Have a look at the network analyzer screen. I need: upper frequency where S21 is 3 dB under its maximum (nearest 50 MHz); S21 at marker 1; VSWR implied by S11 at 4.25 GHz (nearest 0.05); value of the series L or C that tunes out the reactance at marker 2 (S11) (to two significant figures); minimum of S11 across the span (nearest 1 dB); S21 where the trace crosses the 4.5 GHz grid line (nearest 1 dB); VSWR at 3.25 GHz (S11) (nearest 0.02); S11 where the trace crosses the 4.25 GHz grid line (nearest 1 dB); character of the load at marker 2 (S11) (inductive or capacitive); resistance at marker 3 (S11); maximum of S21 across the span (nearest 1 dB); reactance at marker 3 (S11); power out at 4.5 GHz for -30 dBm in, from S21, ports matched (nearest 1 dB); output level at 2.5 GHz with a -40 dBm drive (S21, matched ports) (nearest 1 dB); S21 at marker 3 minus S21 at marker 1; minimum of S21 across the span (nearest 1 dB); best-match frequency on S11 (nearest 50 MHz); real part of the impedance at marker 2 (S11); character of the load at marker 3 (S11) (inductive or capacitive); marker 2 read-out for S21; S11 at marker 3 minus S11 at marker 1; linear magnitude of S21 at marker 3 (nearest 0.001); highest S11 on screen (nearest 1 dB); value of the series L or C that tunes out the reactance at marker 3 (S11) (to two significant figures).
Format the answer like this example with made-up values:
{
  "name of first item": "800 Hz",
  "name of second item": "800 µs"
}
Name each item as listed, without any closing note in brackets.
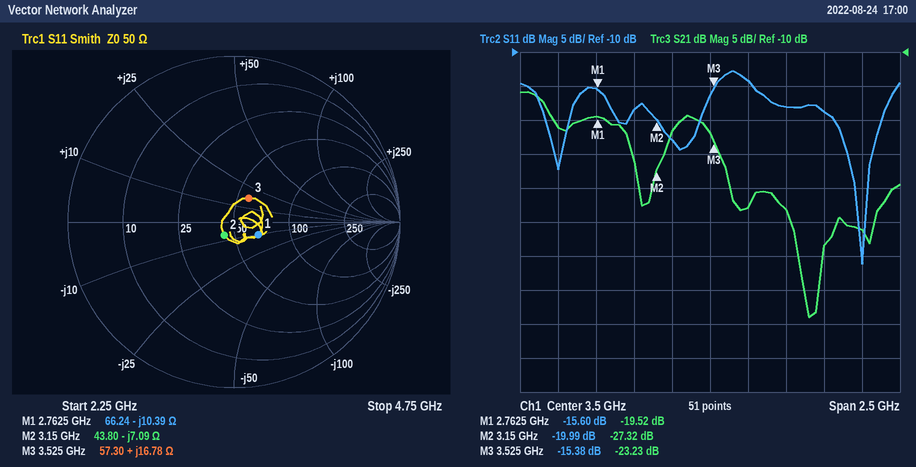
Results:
{
  "upper frequency where S21 is 3 dB under its maximum": "2.45 GHz",
  "S21 at marker 1": "-19.52 dB",
  "VSWR implied by S11 at 4.25 GHz": "1.25",
  "value of the series L or C that tunes out the reactance at marker 2 (S11)": "360 pH",
  "minimum of S11 across the span": "-41 dB",
  "S21 where the trace crosses the 4.5 GHz grid line": "-36 dB",
  "VSWR at 3.25 GHz (S11)": "1.16",
  "S11 where the trace crosses the 4.25 GHz grid line": "-19 dB",
  "character of the load at marker 2 (S11)": "capacitive",
  "resistance at marker 3": "57.30 Ω",
  "maximum of S21 across the span": "-16 dB",
  "reactance at marker 3": "+16.78 Ω",
  "power out at 4.5 GHz for -30 dBm in, from S21, ports matched": "-66 dBm",
  "output level at 2.5 GHz with a -40 dBm drive (S21, matched ports)": "-61 dBm",
  "S21 at marker 3 minus S21 at marker 1": "-3.71 dB",
  "minimum of S21 across the span": "-49 dB",
  "best-match frequency on S11": "4.50 GHz",
  "real part of the impedance at marker 2": "43.80 Ω",
  "character of the load at marker 3 (S11)": "inductive",
  "marker 2 read-out for S21": "-27.32 dB",
  "S11 at marker 3 minus S11 at marker 1": "0.22 dB",
  "linear magnitude of S21 at marker 3": "0.069",
  "highest S11 on screen": "-13 dB",
  "value of the series L or C that tunes out the reactance at marker 3 (S11)": "2.7 pF"
}
